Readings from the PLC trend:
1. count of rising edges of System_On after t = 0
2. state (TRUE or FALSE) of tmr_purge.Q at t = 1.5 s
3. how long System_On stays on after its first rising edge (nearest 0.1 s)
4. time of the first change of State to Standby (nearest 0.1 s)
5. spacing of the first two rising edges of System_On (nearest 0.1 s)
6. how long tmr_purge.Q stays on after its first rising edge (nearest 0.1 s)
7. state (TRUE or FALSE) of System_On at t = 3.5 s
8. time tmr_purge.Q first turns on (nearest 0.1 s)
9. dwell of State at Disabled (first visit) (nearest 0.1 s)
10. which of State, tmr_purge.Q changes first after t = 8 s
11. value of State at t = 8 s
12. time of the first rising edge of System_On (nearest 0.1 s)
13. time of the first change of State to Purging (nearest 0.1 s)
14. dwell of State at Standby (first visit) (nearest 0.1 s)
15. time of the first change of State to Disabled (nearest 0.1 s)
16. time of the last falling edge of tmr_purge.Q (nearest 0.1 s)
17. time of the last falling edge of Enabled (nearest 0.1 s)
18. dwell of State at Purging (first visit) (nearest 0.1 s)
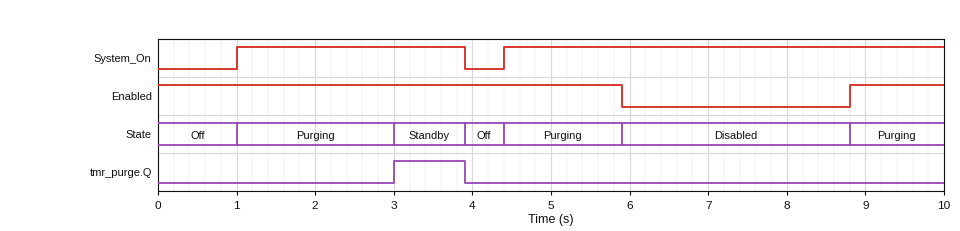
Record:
2
FALSE
2.9 s
3.0 s
3.4 s
0.9 s
TRUE
3.0 s
2.9 s
State
Disabled
1.0 s
1.0 s
0.9 s
5.9 s
3.9 s
5.9 s
2.0 s
